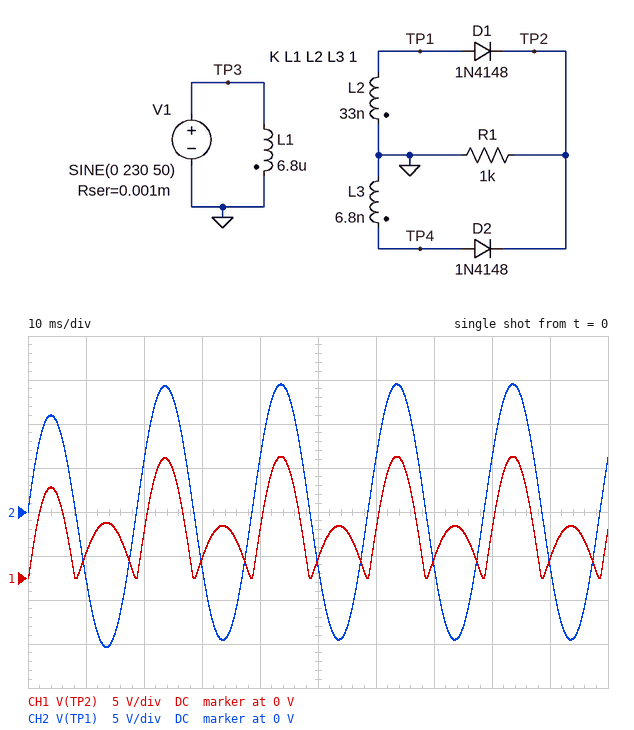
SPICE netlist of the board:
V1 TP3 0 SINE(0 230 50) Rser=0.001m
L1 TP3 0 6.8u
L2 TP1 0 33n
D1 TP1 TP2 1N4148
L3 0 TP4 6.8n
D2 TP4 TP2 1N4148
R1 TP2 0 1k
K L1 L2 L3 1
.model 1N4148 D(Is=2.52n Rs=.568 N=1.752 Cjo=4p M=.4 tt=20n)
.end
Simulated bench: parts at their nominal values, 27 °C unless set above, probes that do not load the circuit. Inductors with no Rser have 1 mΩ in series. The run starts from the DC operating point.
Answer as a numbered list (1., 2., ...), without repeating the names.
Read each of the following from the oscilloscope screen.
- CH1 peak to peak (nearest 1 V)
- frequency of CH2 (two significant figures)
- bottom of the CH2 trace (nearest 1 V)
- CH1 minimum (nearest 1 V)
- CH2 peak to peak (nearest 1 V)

1. 14 V
2. 50 Hz
3. -15 V
4. 0 V
5. 30 V
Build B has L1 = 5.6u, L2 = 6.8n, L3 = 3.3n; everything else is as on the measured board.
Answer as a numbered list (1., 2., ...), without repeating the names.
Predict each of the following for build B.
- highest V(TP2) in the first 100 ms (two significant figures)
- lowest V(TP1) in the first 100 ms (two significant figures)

1. 6.3 V
2. -7.3 V
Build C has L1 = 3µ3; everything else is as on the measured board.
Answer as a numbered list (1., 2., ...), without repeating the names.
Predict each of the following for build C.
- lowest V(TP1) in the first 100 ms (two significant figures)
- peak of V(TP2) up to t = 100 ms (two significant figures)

1. -17 V
2. 16 V
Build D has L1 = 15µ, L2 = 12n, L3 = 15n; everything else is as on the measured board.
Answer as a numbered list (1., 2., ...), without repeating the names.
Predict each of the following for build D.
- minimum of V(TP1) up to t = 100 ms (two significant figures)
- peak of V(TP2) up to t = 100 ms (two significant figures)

1. -6.9 V
2. 7.0 V
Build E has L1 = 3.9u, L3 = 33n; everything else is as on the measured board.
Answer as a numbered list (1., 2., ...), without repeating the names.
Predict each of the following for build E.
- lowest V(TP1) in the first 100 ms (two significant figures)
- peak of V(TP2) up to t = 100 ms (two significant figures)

1. -17 V
2. 16 V
